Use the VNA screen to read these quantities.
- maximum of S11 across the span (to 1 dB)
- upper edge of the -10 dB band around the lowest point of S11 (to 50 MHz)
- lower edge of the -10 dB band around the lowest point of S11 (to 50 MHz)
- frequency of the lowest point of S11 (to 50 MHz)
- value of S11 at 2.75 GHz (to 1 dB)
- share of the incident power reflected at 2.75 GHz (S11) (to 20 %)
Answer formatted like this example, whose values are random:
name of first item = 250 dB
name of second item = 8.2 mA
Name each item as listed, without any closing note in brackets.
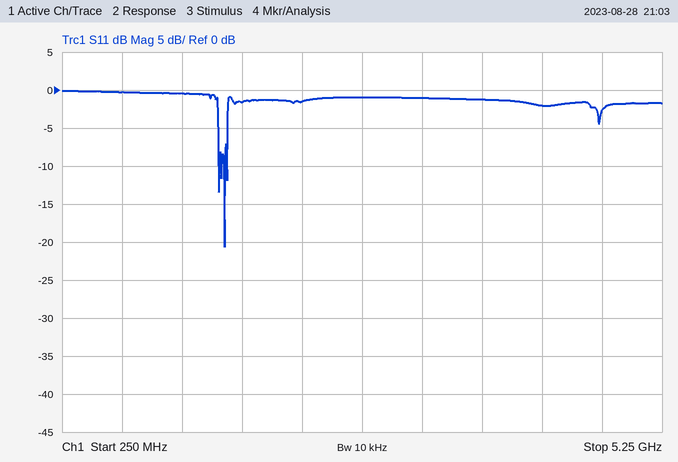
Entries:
maximum of S11 across the span = 0 dB
upper edge of the -10 dB band around the lowest point of S11 = 1.60 GHz
lower edge of the -10 dB band around the lowest point of S11 = 1.60 GHz
frequency of the lowest point of S11 = 1.60 GHz
value of S11 at 2.75 GHz = -1 dB
share of the incident power reflected at 2.75 GHz (S11) = 80 %
